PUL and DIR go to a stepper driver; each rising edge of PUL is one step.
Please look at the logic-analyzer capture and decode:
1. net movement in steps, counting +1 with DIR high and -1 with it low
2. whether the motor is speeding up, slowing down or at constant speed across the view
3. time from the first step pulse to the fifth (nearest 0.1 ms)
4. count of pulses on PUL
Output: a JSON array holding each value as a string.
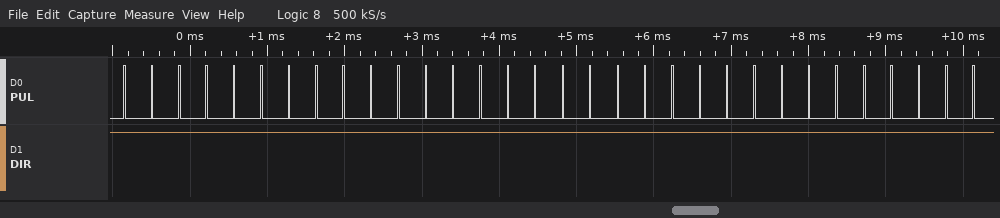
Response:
["+32", "constant speed", "1.4 ms", "32"]
